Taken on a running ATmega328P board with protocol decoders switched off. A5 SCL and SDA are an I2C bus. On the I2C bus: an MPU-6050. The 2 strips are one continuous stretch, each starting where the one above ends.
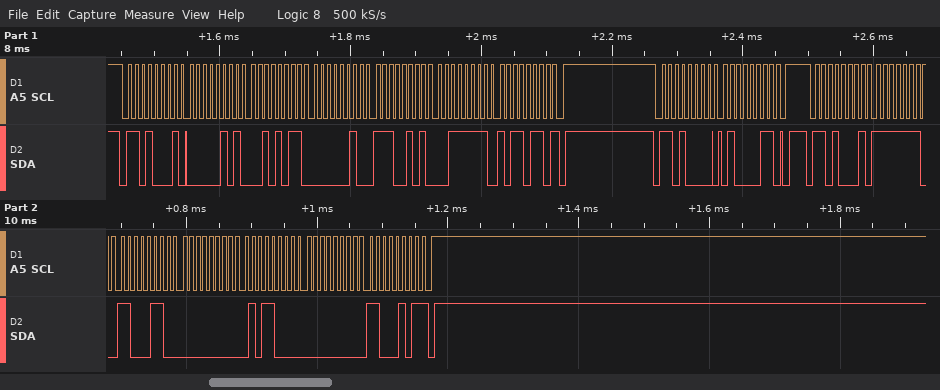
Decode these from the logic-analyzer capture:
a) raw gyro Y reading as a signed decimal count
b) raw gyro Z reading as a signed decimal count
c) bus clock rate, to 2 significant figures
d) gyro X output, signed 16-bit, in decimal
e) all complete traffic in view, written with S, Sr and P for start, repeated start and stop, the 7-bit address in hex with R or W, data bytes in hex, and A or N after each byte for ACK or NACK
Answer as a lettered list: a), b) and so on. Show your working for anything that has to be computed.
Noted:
a) 0x0058 = 88
b) 0x00C5 = 197
c) 100 kHz
d) 0xFEC6 = -314
e) S 68R A 05 A 2B A 02 A E5 A 3F A B6 N P S 68W A 43 A P S 68R A FE A C6 A 00 A 58 A 00 A C5 N P
